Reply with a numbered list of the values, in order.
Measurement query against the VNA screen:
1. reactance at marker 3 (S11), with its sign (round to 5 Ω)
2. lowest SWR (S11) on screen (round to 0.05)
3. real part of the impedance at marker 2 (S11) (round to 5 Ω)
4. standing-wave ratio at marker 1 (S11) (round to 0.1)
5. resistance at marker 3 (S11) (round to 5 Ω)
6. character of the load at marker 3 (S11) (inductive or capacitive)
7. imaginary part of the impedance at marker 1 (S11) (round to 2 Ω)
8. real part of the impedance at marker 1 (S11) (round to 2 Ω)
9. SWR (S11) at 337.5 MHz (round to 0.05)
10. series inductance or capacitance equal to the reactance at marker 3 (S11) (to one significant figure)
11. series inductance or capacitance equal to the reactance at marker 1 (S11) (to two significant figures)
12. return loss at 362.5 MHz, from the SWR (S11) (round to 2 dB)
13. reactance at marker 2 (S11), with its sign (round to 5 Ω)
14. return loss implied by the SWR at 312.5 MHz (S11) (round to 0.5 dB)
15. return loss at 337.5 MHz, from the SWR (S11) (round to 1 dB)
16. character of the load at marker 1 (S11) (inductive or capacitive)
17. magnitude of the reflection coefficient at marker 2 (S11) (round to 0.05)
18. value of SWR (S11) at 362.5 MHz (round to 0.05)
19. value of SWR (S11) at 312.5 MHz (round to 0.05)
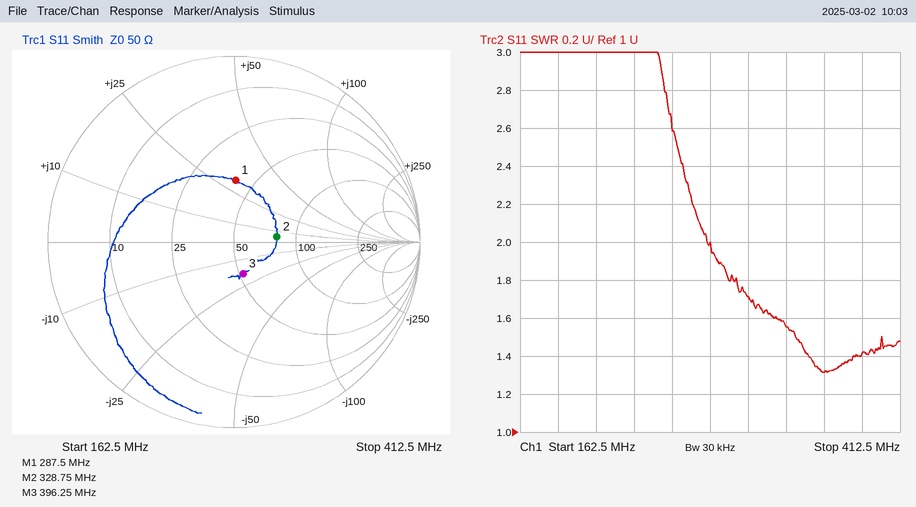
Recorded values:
1. -20 Ω
2. 1.30
3. 80 Ω
4. 2.0
5. 50 Ω
6. capacitive
7. +30 Ω
8. 40 Ω
9. 1.55
10. 20 pF
11. 17 nH
12. 18 dB
13. +5 Ω
14. 11.5 dB
15. 13 dB
16. inductive
17. 0.25
18. 1.30
19. 1.70
